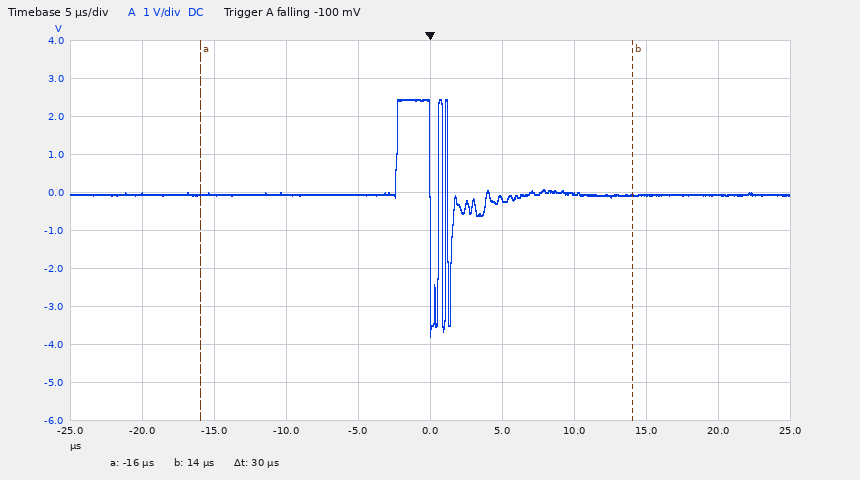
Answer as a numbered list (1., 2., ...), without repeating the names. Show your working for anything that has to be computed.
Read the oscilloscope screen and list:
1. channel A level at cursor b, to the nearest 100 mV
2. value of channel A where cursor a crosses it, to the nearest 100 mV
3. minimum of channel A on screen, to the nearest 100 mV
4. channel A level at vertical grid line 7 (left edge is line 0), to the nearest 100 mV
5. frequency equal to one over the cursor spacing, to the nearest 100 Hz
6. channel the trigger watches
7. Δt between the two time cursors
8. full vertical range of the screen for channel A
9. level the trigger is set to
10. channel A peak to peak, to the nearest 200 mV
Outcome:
1. -100 mV
2. -100 mV
3. -3.8 V
4. 0.0 V
5. 1 / 30 µs ≈ 33.3 kHz
6. channel A
7. 30 µs
8. 10 V
9. -100 mV
10. 6.2 V
